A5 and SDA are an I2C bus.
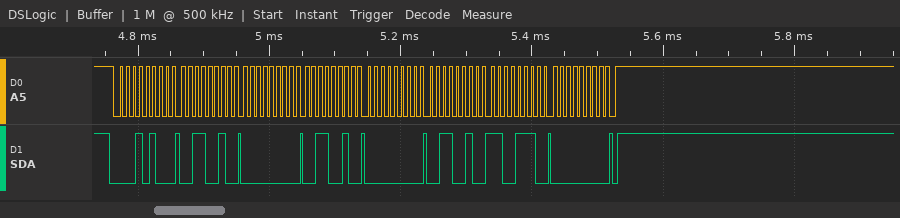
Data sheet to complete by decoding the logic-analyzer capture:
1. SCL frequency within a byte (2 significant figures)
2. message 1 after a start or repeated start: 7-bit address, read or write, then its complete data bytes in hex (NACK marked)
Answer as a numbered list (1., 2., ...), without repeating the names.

1. 100 kHz
2. 0x0A write: 32 00 32 00 32 CE 00
